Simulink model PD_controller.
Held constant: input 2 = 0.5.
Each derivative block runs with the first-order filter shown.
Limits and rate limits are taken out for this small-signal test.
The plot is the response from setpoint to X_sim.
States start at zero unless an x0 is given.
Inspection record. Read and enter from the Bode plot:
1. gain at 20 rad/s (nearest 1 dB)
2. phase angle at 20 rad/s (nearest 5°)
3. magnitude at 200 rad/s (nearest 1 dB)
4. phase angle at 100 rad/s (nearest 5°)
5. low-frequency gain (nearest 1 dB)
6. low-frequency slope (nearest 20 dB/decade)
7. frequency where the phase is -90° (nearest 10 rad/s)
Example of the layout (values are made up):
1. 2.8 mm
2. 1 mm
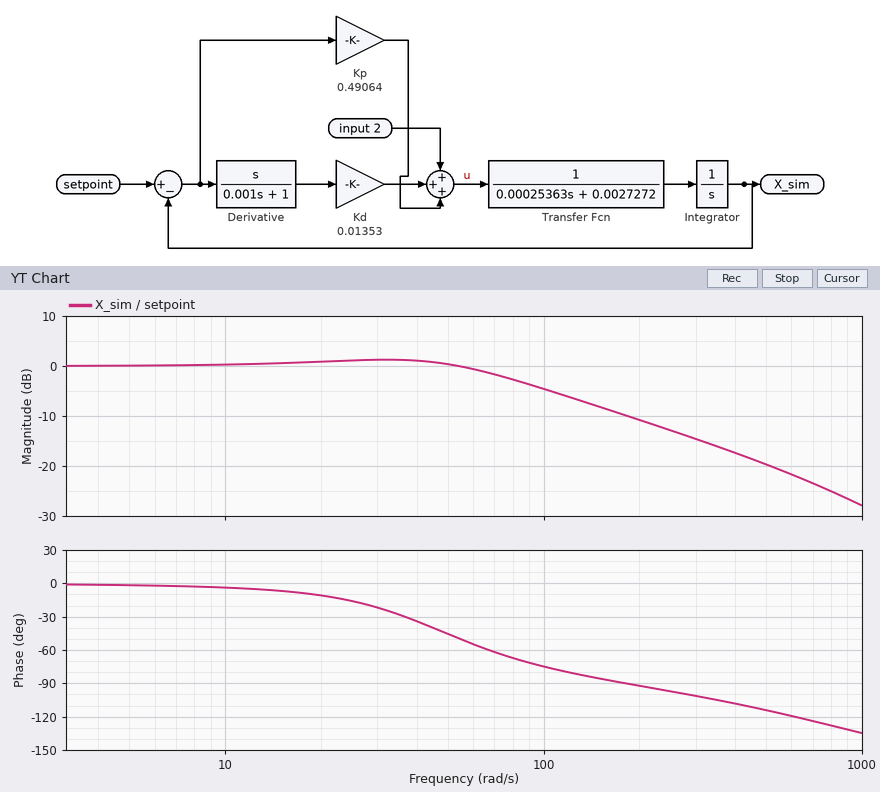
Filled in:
1. 1 dB
2. -10°
3. -11 dB
4. -75°
5. 0 dB
6. 0 dB/decade
7. 180 rad/s
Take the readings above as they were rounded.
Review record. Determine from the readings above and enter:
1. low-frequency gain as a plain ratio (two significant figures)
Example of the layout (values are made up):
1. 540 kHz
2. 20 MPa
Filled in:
1. 1.0
